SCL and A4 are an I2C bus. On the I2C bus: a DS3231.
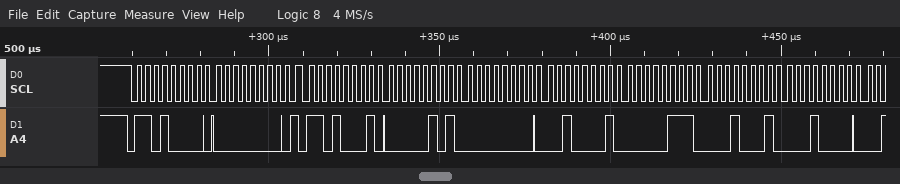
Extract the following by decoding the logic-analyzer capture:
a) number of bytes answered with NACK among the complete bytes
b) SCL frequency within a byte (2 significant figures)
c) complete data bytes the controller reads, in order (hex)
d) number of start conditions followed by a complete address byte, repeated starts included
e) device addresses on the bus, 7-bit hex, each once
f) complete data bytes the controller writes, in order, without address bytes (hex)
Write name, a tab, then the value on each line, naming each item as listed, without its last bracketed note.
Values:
number of bytes answered with NACK among the complete bytes	0
SCL frequency within a byte	400 kHz
complete data bytes the controller reads, in order	05 00 21 07 11 10
number of start conditions followed by a complete address byte, repeated starts included	2
device addresses on the bus, 7-bit hex, each once	0x68
complete data bytes the controller writes, in order, without address bytes	00
